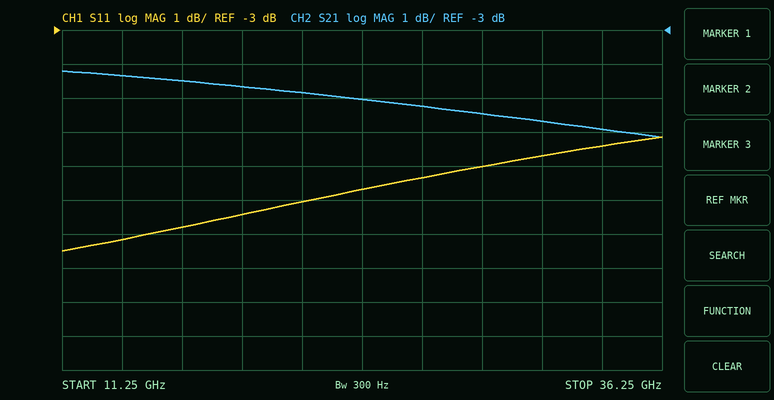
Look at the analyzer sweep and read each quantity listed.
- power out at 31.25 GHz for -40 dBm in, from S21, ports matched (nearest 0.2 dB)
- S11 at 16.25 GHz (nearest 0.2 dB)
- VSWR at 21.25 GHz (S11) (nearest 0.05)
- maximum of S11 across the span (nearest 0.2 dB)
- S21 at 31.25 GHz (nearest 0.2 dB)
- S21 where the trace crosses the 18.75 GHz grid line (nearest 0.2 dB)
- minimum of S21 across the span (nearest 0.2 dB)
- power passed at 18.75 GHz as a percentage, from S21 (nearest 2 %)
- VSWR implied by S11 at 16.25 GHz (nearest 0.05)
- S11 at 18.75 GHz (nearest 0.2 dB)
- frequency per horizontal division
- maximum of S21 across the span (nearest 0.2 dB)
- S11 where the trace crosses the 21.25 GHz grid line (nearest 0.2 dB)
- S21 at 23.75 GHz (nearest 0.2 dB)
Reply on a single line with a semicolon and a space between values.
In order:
-45.6 dBm; -8.8 dB; 2.30; -6.2 dB; -5.6 dB; -4.6 dB; -6.2 dB; 34 %; 2.15; -8.4 dB; 2.5 GHz; -4.2 dB; -8.0 dB; -5.0 dB
